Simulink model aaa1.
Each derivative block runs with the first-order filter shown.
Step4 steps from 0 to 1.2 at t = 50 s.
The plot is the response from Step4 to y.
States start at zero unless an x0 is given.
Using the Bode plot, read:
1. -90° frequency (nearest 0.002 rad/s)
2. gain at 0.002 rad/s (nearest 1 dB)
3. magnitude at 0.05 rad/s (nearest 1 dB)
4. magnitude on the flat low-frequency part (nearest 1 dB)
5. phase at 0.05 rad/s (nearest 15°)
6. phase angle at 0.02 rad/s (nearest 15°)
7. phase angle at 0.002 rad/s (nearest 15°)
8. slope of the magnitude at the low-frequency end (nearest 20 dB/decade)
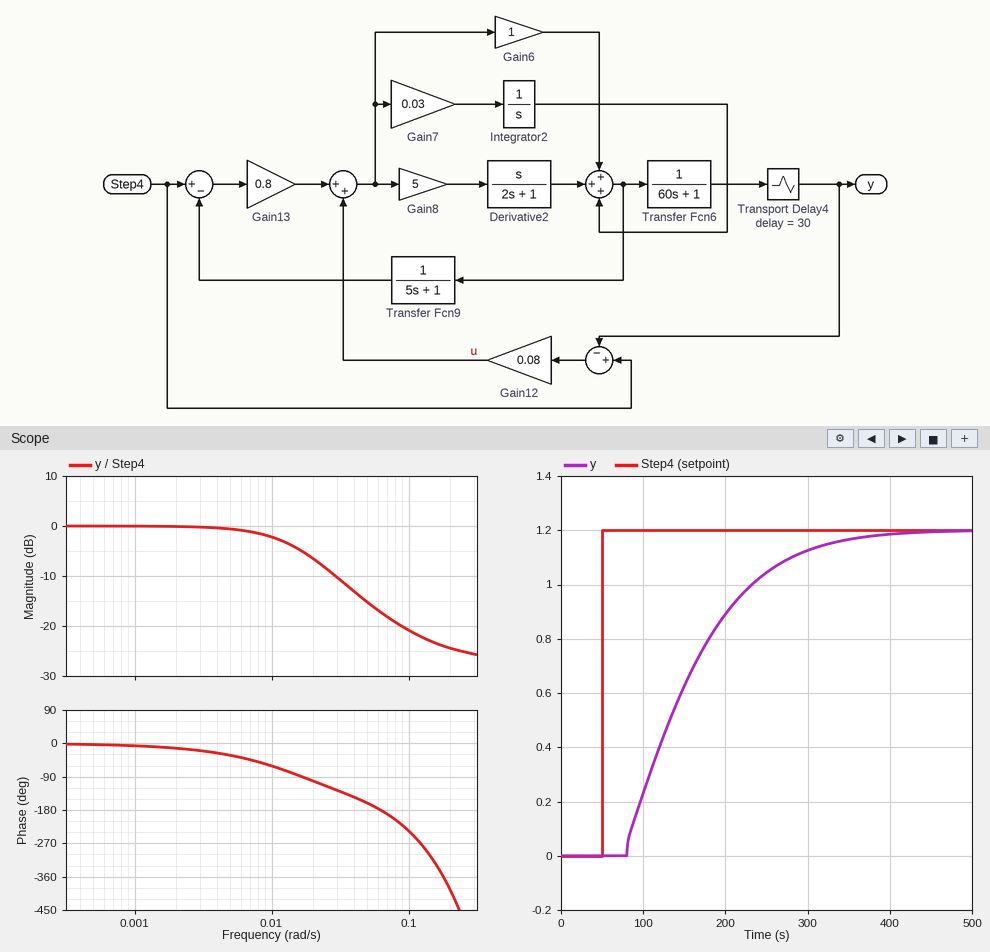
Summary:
0.016 rad/s
0 dB
-15 dB
0 dB
-165°
-105°
-15°
0 dB/decade
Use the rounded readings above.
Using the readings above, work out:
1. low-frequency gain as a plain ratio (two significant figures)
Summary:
1.0
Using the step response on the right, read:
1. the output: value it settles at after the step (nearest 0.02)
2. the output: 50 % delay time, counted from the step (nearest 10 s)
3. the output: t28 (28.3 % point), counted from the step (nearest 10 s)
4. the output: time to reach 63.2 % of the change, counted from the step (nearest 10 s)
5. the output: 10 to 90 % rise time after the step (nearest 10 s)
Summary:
1.20
100 s
60 s
120 s
180 s
